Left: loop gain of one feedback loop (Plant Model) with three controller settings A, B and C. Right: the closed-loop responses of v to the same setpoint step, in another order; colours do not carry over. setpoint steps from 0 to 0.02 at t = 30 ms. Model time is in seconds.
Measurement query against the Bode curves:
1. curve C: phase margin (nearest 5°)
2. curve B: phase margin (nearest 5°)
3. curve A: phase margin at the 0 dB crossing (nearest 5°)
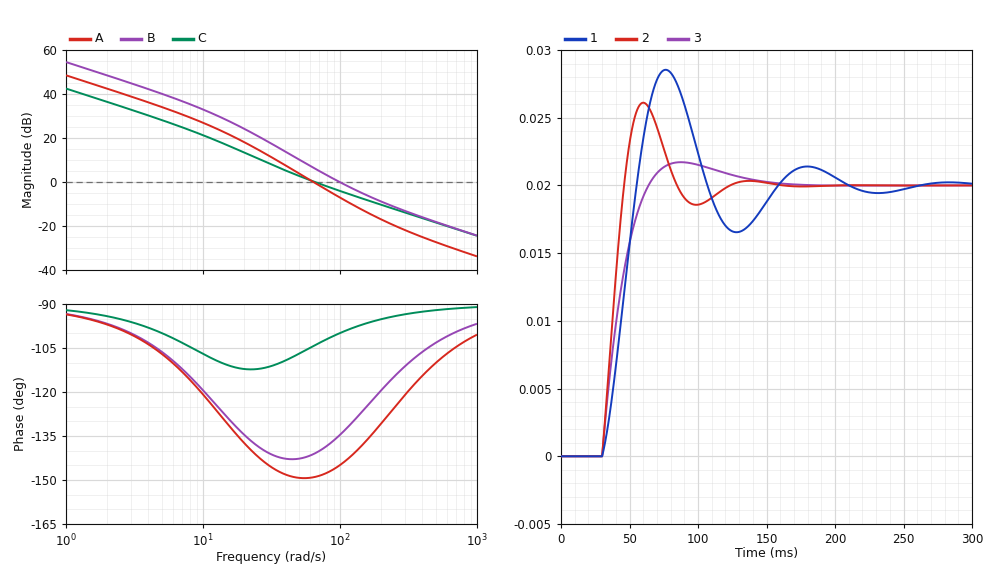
75°
45°
30°
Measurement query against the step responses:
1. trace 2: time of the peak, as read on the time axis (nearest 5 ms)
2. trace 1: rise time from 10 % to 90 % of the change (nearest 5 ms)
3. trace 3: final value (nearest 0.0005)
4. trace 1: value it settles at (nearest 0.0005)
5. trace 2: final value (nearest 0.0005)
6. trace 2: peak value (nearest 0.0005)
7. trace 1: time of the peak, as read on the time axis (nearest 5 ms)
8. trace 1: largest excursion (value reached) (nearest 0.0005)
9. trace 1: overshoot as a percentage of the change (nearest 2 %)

60 ms
20 ms
0.0200
0.0200
0.0200
0.0260
75 ms
0.0285
42 %
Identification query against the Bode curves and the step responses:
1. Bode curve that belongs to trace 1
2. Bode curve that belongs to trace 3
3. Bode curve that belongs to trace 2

A
C
B
